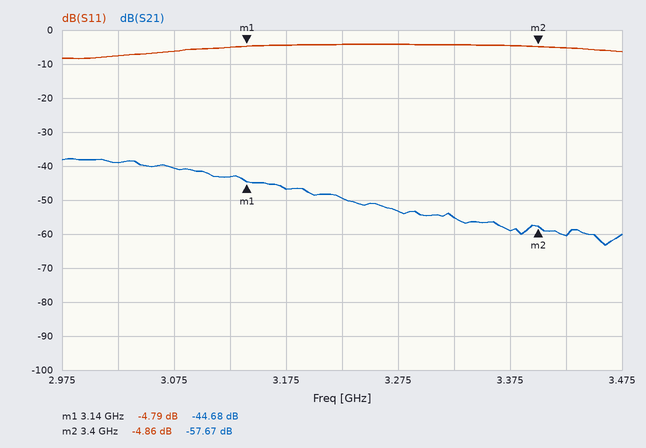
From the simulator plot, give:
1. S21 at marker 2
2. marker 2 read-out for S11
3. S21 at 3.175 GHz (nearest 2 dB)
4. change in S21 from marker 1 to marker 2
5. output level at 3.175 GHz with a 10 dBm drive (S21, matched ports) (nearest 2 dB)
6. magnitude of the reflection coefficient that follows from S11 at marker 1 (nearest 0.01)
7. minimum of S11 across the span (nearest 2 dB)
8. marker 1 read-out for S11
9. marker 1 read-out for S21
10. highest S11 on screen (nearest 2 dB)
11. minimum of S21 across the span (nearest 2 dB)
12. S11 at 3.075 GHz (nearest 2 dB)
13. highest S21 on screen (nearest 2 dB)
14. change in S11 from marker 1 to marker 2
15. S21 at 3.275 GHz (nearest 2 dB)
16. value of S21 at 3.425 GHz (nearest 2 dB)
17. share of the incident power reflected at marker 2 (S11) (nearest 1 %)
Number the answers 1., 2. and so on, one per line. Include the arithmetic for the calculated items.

1. -57.67 dB
2. -4.86 dB
3. -46 dB
4. -57.67 − (-44.68) = -12.99 dB
5. 10 dBm + (-46 dB) = -36 dBm
6. 10^(-4.79/20) ≈ 0.58
7. -8 dB
8. -4.79 dB
9. -44.68 dB
10. -4 dB
11. -64 dB
12. -6 dB
13. -38 dB
14. -4.86 − (-4.79) = -0.07 dB
15. -54 dB
16. -60 dB
17. 10^(-4.86/10) ≈ 33 %
